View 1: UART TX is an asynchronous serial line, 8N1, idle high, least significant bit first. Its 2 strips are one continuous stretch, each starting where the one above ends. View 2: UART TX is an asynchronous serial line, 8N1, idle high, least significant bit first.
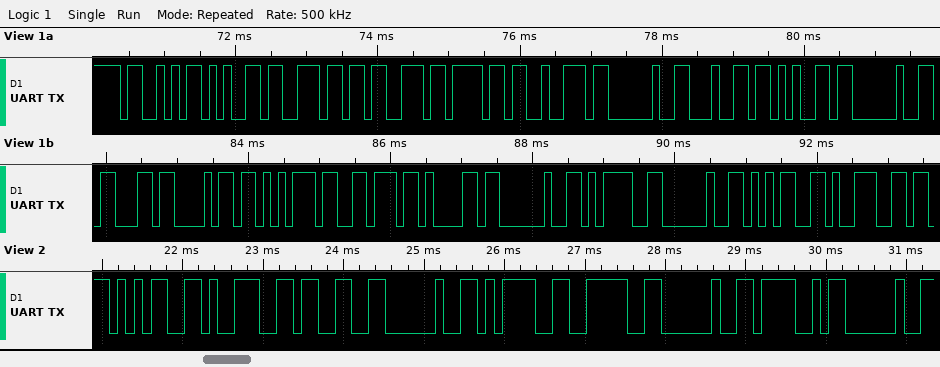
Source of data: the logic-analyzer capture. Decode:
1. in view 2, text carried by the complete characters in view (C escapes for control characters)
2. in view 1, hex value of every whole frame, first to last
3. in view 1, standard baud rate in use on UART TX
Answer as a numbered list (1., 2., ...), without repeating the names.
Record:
1. "593 => O "
2. 53 65 6E 73 6F 72 20 64 65 20 63 68 75 76 61 20 3D 20 35 39
3. 9600 baud
